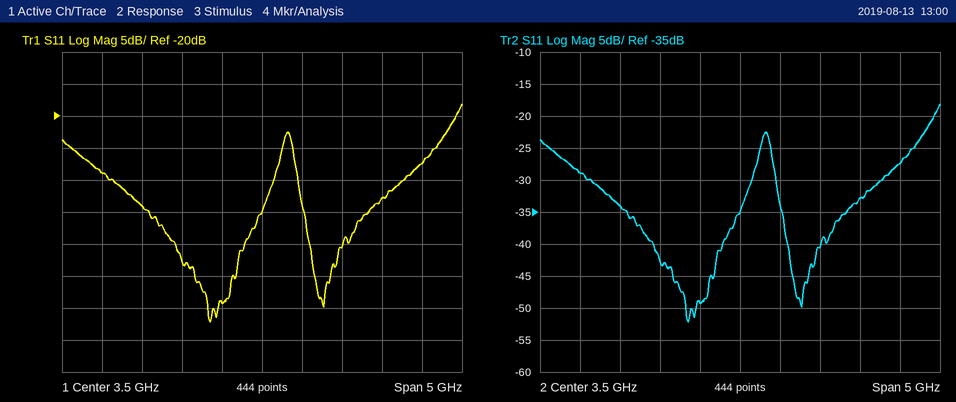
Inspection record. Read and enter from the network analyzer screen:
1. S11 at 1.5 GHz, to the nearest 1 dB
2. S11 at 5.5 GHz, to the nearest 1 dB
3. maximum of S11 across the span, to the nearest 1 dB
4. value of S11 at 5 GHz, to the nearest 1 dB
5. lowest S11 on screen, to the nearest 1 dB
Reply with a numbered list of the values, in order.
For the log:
1. -29 dB
2. -27 dB
3. -18 dB
4. -33 dB
5. -52 dB
